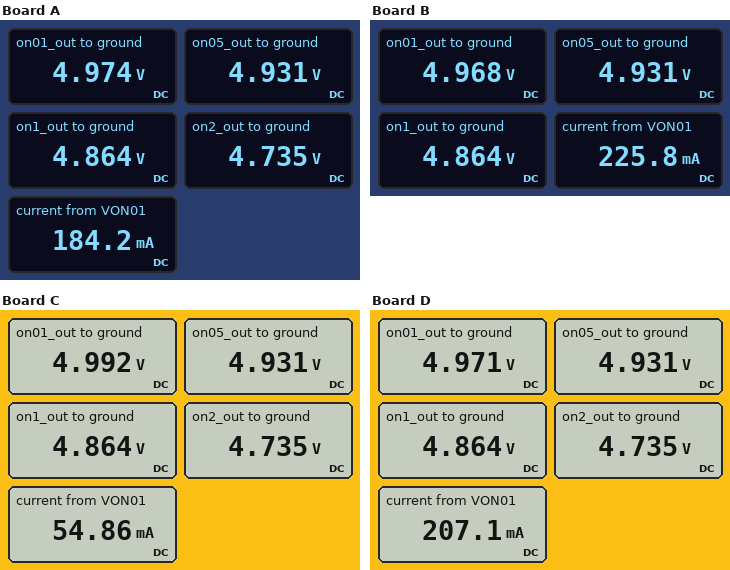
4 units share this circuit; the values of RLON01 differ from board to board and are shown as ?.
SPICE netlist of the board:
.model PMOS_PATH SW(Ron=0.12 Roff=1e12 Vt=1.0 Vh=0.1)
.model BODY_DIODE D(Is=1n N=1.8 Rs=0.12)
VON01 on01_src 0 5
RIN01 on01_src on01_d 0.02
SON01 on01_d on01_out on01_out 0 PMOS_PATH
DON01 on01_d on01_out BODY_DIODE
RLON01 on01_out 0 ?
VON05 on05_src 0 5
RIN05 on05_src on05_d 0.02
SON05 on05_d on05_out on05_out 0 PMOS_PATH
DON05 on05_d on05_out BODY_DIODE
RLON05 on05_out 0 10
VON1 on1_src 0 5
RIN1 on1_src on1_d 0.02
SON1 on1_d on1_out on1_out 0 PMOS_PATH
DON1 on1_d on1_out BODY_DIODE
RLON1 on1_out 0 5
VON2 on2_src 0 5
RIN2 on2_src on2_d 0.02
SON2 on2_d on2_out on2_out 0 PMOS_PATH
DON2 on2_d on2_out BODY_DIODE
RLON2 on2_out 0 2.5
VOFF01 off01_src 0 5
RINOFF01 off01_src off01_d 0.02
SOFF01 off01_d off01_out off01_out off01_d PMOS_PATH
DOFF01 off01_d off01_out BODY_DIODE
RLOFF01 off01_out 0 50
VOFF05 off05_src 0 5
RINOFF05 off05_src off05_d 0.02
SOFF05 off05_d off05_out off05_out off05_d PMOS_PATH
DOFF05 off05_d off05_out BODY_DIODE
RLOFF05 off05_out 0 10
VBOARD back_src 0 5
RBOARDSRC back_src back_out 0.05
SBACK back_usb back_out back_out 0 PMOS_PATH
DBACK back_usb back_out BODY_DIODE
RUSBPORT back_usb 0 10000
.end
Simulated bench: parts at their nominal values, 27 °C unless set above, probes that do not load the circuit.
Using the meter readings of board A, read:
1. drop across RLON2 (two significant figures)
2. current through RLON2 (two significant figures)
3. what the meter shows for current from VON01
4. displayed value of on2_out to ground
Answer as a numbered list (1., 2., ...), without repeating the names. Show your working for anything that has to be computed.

1. 4.735 V = 4.7 V
2. (4.735 V) / 2.5 Ω = 1.9 A
3. 184.2 mA
4. 4.735 V
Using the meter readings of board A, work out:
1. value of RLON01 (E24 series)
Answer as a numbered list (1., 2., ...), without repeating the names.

1. 27 Ω
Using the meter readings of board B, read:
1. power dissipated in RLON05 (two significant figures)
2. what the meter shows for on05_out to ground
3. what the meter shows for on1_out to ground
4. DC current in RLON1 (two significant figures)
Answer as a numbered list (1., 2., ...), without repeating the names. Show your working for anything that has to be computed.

1. (4.931 V)^2 / 10 Ω = 2.4 W
2. 4.931 V
3. 4.864 V
4. (4.864 V) / 5 Ω = 970 mA
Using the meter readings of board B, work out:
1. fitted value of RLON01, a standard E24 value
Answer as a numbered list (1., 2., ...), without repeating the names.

1. 22 Ω
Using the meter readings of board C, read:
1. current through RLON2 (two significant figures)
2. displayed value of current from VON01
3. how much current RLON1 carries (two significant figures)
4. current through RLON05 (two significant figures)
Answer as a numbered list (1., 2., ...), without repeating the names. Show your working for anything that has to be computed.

1. (4.735 V) / 2.5 Ω = 1.9 A
2. 54.86 mA
3. (4.864 V) / 5 Ω = 970 mA
4. (4.931 V) / 10 Ω = 490 mA
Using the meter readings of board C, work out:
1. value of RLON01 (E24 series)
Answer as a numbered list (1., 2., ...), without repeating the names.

1. 91 Ω
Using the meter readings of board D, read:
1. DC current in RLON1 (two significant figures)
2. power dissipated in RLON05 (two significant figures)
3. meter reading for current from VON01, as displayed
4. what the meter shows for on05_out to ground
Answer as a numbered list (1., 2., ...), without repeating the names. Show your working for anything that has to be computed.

1. (4.864 V) / 5 Ω = 970 mA
2. (4.931 V)^2 / 10 Ω = 2.4 W
3. 207.1 mA
4. 4.931 V
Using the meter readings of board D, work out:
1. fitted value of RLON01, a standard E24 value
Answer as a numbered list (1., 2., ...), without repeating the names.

1. 24 Ω
